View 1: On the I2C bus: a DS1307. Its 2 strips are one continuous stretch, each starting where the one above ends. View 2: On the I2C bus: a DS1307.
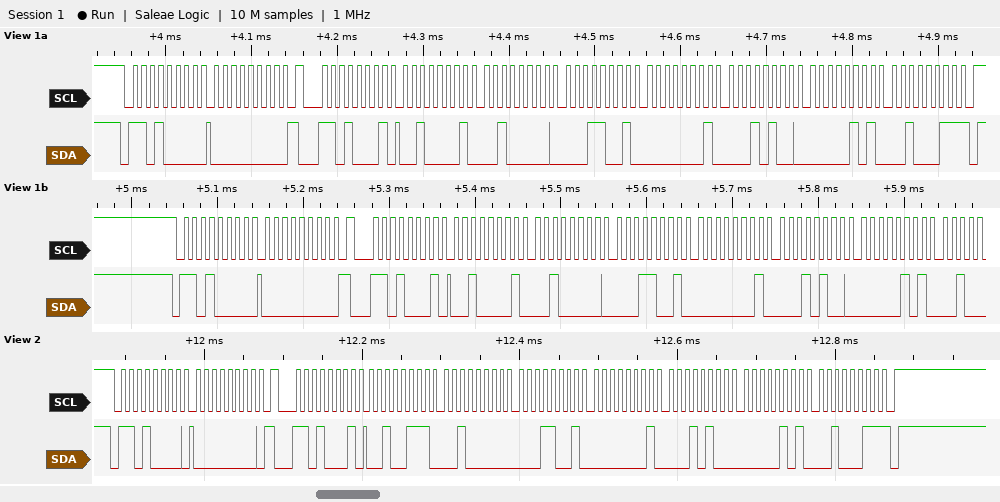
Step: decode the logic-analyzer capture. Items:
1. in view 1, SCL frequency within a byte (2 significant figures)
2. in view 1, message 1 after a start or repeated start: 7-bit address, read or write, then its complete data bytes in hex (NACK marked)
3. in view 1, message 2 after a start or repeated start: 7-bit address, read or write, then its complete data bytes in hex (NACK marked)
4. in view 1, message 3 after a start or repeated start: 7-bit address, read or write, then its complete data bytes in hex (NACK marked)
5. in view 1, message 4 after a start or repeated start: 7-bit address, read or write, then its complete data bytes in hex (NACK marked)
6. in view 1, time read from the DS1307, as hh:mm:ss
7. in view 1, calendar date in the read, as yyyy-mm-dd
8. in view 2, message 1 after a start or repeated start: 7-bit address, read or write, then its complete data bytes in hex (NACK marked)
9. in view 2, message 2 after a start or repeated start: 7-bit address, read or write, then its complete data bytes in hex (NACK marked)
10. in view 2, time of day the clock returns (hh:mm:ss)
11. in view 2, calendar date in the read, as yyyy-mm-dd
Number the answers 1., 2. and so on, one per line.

1. 100 kHz
2. 0x68 write: 00
3. 0x68 read: 21 20 19 01 14 05 23 NACK
4. 0x68 write: 00
5. 0x68 read: 21 20 19 01 14 05
6. 19:20:21
7. 2023-05-14
8. 0x68 write: 00
9. 0x68 read: 27 20 19 01 14 05 23 NACK
10. 19:20:27
11. 2023-05-14
